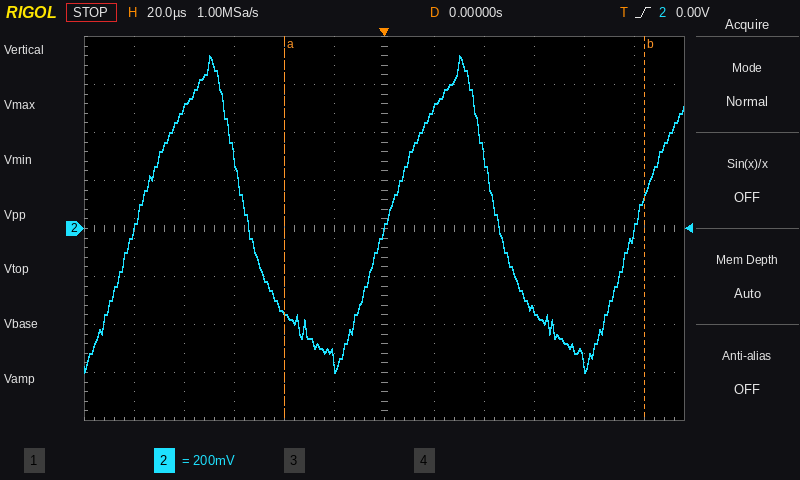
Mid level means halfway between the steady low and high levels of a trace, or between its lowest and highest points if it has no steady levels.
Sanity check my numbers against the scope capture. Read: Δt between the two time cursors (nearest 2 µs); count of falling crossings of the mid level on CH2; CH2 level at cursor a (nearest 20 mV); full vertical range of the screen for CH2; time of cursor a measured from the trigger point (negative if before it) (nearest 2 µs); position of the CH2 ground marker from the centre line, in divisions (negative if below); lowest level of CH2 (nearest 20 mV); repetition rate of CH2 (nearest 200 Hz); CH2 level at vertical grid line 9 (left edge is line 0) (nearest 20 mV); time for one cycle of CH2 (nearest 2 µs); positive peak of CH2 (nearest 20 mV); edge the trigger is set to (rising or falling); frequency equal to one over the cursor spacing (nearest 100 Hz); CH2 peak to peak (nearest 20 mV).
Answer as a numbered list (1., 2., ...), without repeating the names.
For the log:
1. 144 µs
2. 2
3. -360 mV
4. 1.6 V
5. -40 µs
6. 0.0 div
7. -600 mV
8. 10.0 kHz
9. -340 mV
10. 100 µs
11. 720 mV
12. rising
13. 6.9 kHz
14. 1.32 V
